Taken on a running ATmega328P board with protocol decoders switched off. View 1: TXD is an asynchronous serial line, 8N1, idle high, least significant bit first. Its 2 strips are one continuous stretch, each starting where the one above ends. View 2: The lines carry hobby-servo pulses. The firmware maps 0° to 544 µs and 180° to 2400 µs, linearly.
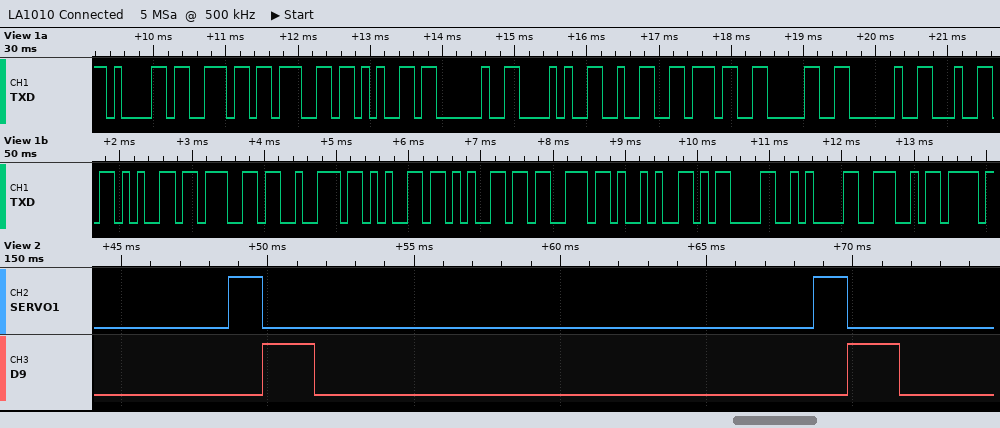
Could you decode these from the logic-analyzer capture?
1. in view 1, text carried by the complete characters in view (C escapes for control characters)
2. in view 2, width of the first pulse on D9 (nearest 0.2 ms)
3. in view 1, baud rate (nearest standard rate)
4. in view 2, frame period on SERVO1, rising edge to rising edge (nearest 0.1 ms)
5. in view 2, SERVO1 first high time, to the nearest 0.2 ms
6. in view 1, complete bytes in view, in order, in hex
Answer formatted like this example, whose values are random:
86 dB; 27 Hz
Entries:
"ange (270 degrees)\r\nN"; 1.8 ms; 9600 baud; 20.0 ms; 1.2 ms; 0x61 0x6E 0x67 0x65 0x20 0x28 0x32 0x37 0x30 0x20 0x64 0x65 0x67 0x72 0x65 0x65 0x73 0x29 0x0D 0x0A 0x4E
